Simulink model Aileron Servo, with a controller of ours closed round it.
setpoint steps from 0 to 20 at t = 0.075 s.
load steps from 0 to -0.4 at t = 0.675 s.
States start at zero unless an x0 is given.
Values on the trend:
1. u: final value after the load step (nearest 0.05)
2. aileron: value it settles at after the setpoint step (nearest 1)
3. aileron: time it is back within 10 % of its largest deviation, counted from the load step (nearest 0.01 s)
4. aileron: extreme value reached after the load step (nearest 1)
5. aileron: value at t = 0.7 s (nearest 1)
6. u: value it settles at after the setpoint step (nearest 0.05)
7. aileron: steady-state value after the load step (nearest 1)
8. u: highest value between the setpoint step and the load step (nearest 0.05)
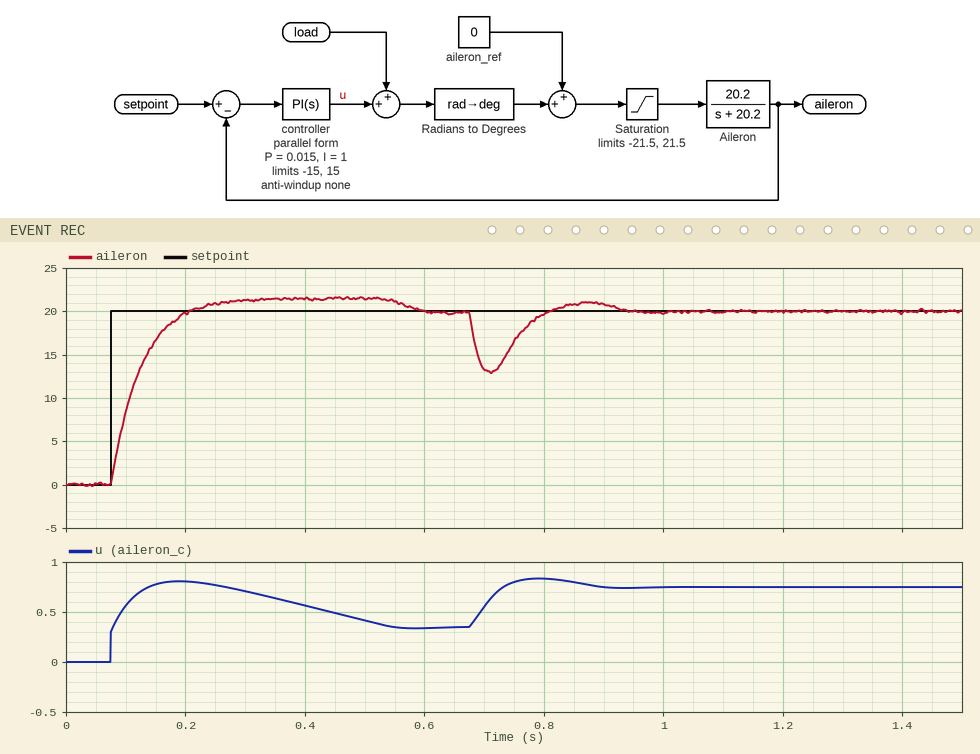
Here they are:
0.75
20
0.23 s
13
13
0.35
20
0.80
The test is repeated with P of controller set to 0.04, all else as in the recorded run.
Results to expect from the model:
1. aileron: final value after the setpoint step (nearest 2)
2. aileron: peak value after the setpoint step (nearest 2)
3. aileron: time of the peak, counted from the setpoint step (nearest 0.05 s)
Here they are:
20
22
0.40 s
